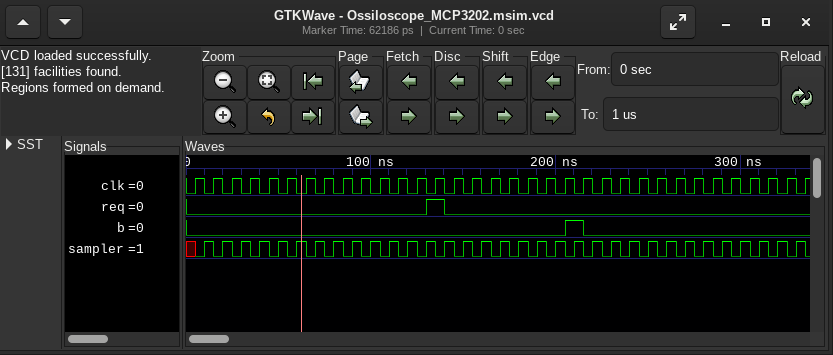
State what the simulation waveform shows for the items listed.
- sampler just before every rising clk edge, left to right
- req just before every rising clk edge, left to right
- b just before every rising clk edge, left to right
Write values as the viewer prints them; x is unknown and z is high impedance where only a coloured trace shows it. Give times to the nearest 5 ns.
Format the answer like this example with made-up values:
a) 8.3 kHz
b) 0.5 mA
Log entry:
a) x 1 1 1 1 1 1 1 1 1 1 1 1 1 1 1 1 1 1 1 1 1 1 1 1 1 1 1 1 1 1 1 1 1
b) 0 0 0 0 0 0 0 0 0 0 0 0 0 1 0 0 0 0 0 0 0 0 0 0 0 0 0 0 0 0 0 0 0 0
c) 0 0 0 0 0 0 0 0 0 0 0 0 0 0 0 0 0 0 0 0 0 1 0 0 0 0 0 0 0 0 0 0 0 0
